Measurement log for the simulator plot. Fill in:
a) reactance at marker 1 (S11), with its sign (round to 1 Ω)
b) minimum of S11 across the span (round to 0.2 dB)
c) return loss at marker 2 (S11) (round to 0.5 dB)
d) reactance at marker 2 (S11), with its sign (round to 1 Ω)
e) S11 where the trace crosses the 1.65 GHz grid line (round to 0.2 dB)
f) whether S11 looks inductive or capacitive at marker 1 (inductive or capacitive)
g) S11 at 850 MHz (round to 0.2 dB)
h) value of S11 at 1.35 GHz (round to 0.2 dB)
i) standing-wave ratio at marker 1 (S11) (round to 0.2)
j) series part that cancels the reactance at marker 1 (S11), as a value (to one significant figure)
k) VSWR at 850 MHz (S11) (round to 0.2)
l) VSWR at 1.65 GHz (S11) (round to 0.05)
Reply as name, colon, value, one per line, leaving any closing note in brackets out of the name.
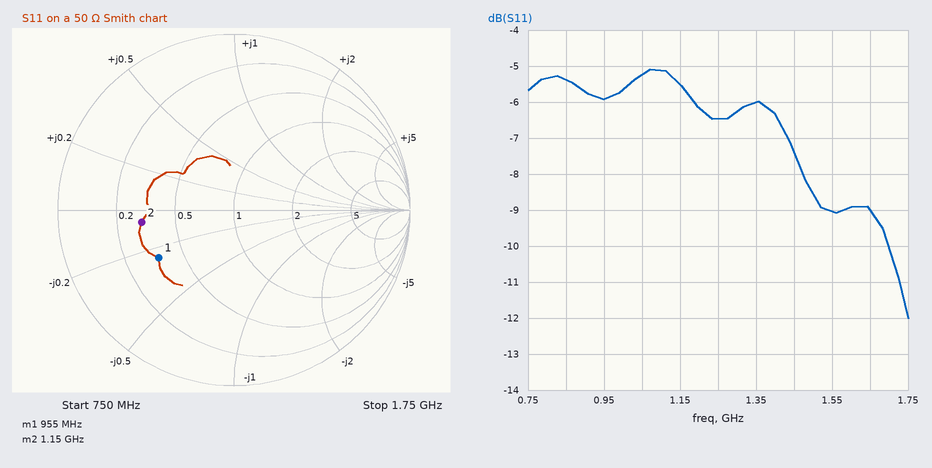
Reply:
reactance at marker 1 (S11), with its sign: -13 Ω
minimum of S11 across the span: -12.0 dB
return loss at marker 2 (S11): 5.5 dB
reactance at marker 2 (S11), with its sign: -3 Ω
S11 where the trace crosses the 1.65 GHz grid line: -9.0 dB
whether S11 looks inductive or capacitive at marker 1: capacitive
S11 at 850 MHz: -5.4 dB
value of S11 at 1.35 GHz: -6.0 dB
standing-wave ratio at marker 1 (S11): 3.0
series part that cancels the reactance at marker 1 (S11), as a value: 2 nH
VSWR at 850 MHz (S11): 3.4
VSWR at 1.65 GHz (S11): 2.10
